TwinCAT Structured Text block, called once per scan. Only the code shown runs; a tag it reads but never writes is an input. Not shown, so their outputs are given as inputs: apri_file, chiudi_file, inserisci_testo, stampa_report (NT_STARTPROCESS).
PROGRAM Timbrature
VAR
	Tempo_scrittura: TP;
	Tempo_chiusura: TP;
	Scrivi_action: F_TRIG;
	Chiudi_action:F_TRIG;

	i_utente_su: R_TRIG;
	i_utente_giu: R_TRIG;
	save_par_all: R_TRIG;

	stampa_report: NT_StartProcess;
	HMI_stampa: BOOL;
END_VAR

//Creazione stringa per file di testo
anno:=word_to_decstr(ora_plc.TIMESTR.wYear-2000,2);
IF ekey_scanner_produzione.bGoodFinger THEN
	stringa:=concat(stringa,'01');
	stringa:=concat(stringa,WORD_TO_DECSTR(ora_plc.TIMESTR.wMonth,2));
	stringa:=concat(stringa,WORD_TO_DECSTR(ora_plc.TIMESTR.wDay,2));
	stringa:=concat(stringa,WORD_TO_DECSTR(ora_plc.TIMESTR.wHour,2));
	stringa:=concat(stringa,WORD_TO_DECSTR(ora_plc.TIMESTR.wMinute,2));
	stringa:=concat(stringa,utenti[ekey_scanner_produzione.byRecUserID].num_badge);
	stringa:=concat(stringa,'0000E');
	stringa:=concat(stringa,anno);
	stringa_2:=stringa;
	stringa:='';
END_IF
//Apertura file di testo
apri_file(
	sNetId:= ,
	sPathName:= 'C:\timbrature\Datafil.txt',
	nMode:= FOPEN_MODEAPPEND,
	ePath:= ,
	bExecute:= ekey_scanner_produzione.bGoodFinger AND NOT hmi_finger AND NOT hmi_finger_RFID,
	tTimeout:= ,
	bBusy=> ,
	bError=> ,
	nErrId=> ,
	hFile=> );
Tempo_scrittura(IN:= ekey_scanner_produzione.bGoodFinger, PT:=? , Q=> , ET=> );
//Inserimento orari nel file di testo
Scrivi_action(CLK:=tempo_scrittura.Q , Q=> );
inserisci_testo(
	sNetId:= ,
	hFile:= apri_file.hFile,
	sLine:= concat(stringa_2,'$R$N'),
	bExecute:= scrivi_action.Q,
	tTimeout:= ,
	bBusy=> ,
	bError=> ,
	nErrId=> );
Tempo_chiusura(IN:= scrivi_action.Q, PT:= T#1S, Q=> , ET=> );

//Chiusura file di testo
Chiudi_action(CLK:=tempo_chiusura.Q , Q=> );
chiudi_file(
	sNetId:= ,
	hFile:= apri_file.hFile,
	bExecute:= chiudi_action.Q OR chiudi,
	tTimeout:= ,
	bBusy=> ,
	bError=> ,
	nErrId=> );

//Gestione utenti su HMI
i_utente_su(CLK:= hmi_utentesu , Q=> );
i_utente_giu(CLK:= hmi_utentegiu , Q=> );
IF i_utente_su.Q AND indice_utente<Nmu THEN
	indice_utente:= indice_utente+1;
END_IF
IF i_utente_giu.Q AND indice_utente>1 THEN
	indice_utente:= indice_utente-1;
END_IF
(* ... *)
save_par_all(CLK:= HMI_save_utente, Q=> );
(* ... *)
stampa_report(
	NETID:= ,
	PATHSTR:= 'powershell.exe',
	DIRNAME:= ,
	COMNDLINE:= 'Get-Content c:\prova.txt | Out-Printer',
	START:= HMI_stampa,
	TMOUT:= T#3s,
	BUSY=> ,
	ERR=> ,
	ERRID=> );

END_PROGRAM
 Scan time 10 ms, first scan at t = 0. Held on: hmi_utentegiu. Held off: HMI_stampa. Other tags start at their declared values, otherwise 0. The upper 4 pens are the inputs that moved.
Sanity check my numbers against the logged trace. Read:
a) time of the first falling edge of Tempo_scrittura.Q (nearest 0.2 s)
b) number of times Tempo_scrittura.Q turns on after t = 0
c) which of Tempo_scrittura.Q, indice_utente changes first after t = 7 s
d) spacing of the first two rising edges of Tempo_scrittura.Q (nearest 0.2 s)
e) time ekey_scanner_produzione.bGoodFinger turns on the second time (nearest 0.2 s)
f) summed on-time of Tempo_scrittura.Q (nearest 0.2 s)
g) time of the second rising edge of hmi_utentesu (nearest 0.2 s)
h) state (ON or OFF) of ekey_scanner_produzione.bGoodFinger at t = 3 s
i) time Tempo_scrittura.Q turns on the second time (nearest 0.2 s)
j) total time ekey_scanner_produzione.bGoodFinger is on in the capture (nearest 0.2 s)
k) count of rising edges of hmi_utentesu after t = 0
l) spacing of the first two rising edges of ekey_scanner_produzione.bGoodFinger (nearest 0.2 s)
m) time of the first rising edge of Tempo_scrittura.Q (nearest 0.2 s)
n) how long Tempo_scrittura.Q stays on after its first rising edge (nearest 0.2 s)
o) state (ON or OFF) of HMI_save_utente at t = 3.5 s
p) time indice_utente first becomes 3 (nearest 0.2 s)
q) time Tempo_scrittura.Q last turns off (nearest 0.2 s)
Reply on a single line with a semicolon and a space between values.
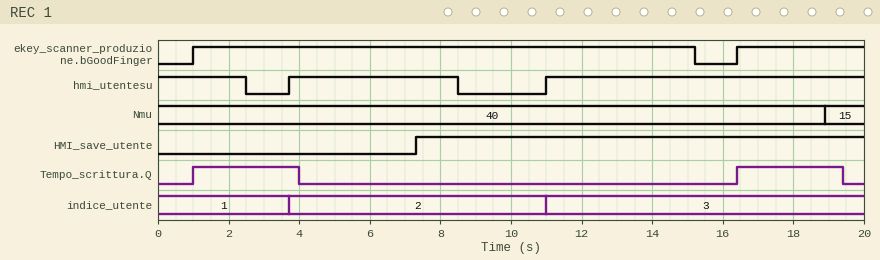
4.0 s; 2; indice_utente; 15.4 s; 16.4 s; 6.0 s; 11.0 s; ON; 16.4 s; 17.8 s; 2; 15.4 s; 1.0 s; 3.0 s; OFF; 11.0 s; 19.4 s
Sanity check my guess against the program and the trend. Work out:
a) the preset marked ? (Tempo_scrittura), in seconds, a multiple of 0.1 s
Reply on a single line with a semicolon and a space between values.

3.0 s
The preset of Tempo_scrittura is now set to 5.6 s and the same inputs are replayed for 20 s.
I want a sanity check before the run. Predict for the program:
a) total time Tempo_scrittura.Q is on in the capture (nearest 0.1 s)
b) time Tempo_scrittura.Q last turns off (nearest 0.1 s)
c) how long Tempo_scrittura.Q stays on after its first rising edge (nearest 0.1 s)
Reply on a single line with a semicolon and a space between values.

9.2 s; 6.6 s; 5.6 s
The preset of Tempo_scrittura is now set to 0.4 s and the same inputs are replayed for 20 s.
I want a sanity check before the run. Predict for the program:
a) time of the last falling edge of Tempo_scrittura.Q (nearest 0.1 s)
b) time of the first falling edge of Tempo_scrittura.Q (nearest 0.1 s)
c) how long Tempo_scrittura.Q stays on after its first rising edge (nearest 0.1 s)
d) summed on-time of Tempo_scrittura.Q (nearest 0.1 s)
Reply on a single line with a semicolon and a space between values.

16.8 s; 1.4 s; 0.4 s; 0.8 s
